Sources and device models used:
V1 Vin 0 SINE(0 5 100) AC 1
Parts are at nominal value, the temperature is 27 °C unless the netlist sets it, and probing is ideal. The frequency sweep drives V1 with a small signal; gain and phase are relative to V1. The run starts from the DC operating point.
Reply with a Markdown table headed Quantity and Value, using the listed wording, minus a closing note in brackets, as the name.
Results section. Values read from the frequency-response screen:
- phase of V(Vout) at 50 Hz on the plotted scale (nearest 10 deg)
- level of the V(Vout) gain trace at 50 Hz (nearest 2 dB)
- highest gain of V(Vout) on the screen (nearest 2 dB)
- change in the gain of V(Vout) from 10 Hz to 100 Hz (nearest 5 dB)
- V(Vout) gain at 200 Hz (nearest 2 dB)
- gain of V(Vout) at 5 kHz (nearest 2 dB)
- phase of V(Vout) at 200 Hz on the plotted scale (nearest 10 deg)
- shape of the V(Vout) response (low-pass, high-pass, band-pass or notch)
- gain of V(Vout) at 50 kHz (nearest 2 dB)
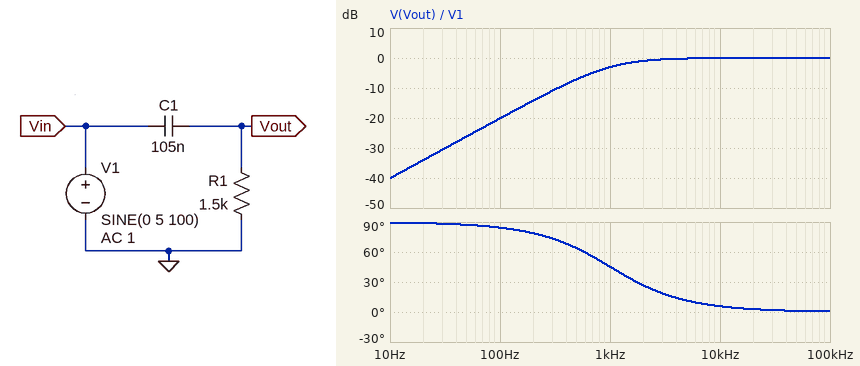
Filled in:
| Quantity | Value |
|---|---|
| phase of V(Vout) at 50 Hz on the plotted scale | 90 deg |
| level of the V(Vout) gain trace at 50 Hz | -26 dB |
| highest gain of V(Vout) on the screen | 0 dB |
| change in the gain of V(Vout) from 10 Hz to 100 Hz | 20 dB |
| V(Vout) gain at 200 Hz | -14 dB |
| gain of V(Vout) at 5 kHz | 0 dB |
| phase of V(Vout) at 200 Hz on the plotted scale | 80 deg |
| shape of the V(Vout) response | high-pass |
| gain of V(Vout) at 50 kHz | 0 dB |
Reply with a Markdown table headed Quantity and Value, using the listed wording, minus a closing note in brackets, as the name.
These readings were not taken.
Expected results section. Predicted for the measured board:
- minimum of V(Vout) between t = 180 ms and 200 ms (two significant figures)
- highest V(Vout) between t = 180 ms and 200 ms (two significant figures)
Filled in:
| Quantity | Value |
|---|---|
| minimum of V(Vout) between t = 180 ms and 200 ms | -490 mV |
| highest V(Vout) between t = 180 ms and 200 ms | 490 mV |
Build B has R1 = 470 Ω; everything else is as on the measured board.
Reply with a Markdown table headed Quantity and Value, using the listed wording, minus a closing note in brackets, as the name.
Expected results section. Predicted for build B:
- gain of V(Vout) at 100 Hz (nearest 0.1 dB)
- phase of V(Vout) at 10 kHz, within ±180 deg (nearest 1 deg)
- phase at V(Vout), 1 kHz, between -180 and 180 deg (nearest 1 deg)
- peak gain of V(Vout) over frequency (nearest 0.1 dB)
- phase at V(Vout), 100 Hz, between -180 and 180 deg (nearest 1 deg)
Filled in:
| Quantity | Value |
|---|---|
| gain of V(Vout) at 100 Hz | -30.2 dB |
| phase of V(Vout) at 10 kHz, within ±180 deg | 18 deg |
| phase at V(Vout), 1 kHz, between -180 and 180 deg | 73 deg |
| peak gain of V(Vout) over frequency | 0 dB |
| phase at V(Vout), 100 Hz, between -180 and 180 deg | 88 deg |
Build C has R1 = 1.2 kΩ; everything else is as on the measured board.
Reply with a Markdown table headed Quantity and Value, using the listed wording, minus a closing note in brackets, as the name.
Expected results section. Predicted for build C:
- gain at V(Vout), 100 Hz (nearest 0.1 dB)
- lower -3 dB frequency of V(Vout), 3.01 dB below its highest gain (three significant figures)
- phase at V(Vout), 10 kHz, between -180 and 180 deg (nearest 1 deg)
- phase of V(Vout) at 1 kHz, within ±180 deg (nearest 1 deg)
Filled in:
| Quantity | Value |
|---|---|
| gain at V(Vout), 100 Hz | -22.1 dB |
| lower -3 dB frequency of V(Vout), 3.01 dB below its highest gain | 1.26 kHz |
| phase at V(Vout), 10 kHz, between -180 and 180 deg | 7 deg |
| phase of V(Vout) at 1 kHz, within ±180 deg | 52 deg |
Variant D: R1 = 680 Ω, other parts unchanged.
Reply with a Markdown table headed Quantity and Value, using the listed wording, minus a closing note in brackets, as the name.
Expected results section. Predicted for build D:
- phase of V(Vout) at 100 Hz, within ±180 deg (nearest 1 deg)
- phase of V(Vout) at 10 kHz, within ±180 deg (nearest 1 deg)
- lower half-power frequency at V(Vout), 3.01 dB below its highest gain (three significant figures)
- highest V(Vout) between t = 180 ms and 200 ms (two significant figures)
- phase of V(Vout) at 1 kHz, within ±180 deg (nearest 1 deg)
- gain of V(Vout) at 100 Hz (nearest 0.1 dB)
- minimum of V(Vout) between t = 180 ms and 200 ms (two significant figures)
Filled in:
| Quantity | Value |
|---|---|
| phase of V(Vout) at 100 Hz, within ±180 deg | 87 deg |
| phase of V(Vout) at 10 kHz, within ±180 deg | 13 deg |
| lower half-power frequency at V(Vout), 3.01 dB below its highest gain | 2.23 kHz |
| highest V(Vout) between t = 180 ms and 200 ms | 220 mV |
| phase of V(Vout) at 1 kHz, within ±180 deg | 66 deg |
| gain of V(Vout) at 100 Hz | -27.0 dB |
| minimum of V(Vout) between t = 180 ms and 200 ms | -220 mV |
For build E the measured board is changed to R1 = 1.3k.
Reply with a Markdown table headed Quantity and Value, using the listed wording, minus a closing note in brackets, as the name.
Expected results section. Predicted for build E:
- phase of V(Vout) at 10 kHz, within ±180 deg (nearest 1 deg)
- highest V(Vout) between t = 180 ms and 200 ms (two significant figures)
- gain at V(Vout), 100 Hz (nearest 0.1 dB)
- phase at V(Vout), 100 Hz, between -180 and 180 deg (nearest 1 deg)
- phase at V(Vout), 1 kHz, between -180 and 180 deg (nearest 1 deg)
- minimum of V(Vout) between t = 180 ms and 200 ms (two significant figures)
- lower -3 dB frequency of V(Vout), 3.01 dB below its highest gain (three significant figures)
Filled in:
| Quantity | Value |
|---|---|
| phase of V(Vout) at 10 kHz, within ±180 deg | 7 deg |
| highest V(Vout) between t = 180 ms and 200 ms | 430 mV |
| gain at V(Vout), 100 Hz | -21.4 dB |
| phase at V(Vout), 100 Hz, between -180 and 180 deg | 85 deg |
| phase at V(Vout), 1 kHz, between -180 and 180 deg | 49 deg |
| minimum of V(Vout) between t = 180 ms and 200 ms | -430 mV |
| lower -3 dB frequency of V(Vout), 3.01 dB below its highest gain | 1.17 kHz |
